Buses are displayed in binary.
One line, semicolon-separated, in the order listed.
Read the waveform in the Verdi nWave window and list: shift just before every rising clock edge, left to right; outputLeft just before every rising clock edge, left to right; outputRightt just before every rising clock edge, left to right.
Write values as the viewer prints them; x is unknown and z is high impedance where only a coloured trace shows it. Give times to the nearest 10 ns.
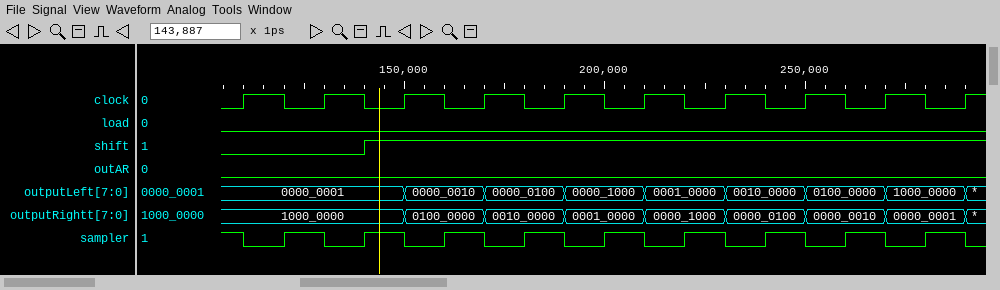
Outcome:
0 0 1 1 1 1 1 1 1 1; 0000_0001, 0000_0001, 0000_0001, 0000_0010, 0000_0100, 0000_1000, 0001_0000, 0010_0000, 0100_0000, 1000_0000; 1000_0000, 1000_0000, 1000_0000, 0100_0000, 0010_0000, 0001_0000, 0000_1000, 0000_0100, 0000_0010, 0000_0001
